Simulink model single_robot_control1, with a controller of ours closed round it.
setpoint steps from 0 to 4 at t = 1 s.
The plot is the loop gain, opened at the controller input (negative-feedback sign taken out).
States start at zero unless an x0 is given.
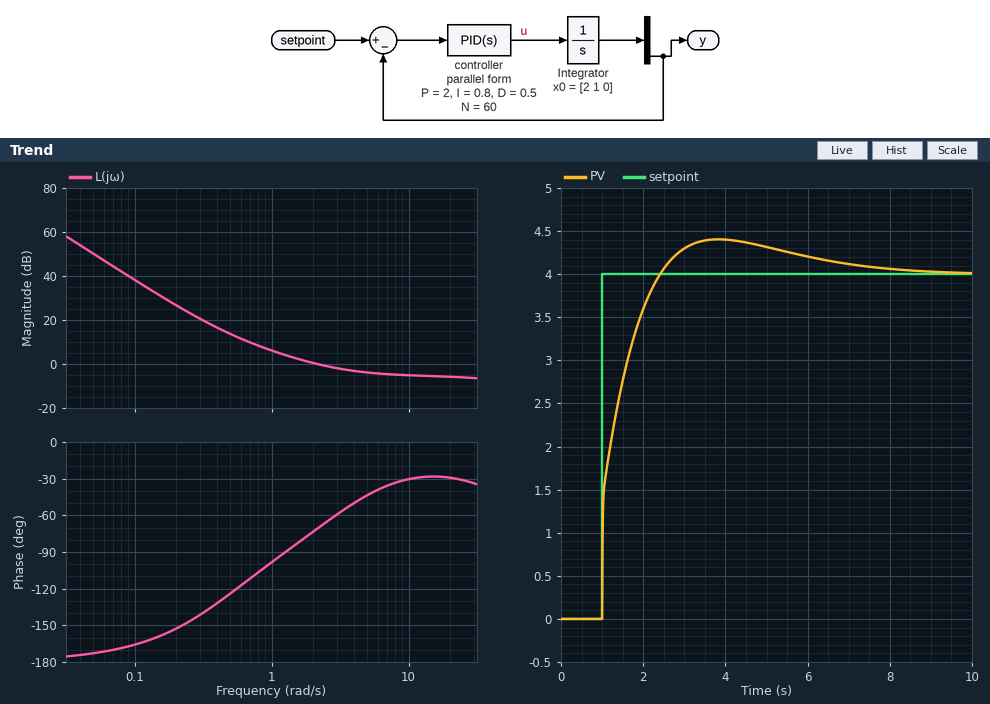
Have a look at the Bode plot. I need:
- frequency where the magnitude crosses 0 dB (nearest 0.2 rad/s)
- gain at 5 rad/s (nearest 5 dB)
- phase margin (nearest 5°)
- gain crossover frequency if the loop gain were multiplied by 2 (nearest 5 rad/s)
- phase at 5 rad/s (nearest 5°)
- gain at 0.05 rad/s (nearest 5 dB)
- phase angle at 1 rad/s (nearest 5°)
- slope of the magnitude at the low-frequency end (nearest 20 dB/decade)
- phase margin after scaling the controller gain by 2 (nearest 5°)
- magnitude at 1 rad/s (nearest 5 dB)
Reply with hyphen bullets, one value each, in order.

- 2.2 rad/s
- -5 dB
- 110°
- 25 rad/s
- -45°
- 50 dB
- -100°
- -40 dB/decade
- 150°
- 5 dB
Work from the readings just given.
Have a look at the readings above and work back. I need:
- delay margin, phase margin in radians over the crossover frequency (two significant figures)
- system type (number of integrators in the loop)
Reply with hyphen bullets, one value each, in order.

- 0.87 s
- 2
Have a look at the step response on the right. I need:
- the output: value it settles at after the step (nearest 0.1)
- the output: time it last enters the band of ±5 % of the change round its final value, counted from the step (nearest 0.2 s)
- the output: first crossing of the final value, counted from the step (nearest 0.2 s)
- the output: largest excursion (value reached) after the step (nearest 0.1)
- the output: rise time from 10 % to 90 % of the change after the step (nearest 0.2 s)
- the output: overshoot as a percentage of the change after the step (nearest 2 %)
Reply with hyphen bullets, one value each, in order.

- 4.0
- 5.0 s
- 1.4 s
- 4.4
- 1.0 s
- 10 %
